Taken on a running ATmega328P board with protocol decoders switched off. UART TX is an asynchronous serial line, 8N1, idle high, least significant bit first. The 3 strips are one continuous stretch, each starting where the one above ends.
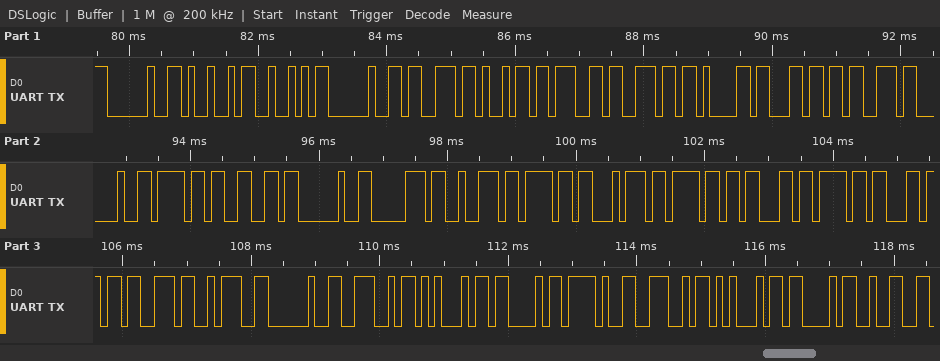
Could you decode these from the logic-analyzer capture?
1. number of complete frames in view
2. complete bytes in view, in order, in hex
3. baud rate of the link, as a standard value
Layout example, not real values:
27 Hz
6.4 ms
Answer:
34
20 49 52 20 73 69 67 6E 61 6C 73 20 6F 66 20 70 72 6F 74 6F 63 6F 6C 73 3A 20 4E 45 43 2F 4E 45 43 32
9600 baud
